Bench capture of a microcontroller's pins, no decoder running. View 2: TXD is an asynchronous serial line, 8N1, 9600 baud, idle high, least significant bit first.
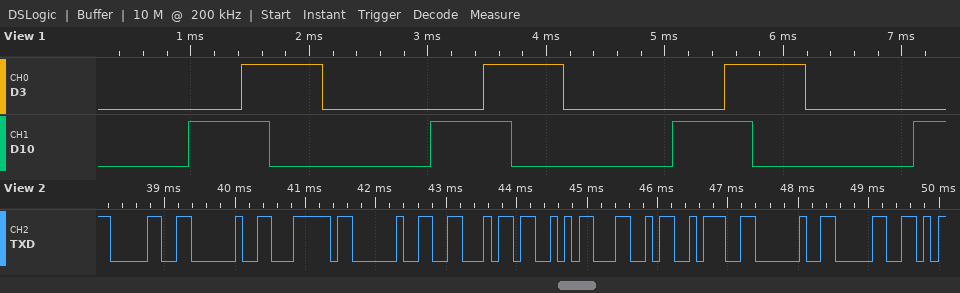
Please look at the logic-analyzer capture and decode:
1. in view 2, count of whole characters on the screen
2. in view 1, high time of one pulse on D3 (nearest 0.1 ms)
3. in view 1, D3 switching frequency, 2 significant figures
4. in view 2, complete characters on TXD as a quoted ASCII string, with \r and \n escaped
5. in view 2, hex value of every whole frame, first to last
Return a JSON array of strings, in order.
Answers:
["10", "0.7 ms", "490 Hz", "\"0 | FSL: 0\"", "30 20 7C 20 46 53 4C 3A 20 30"]
